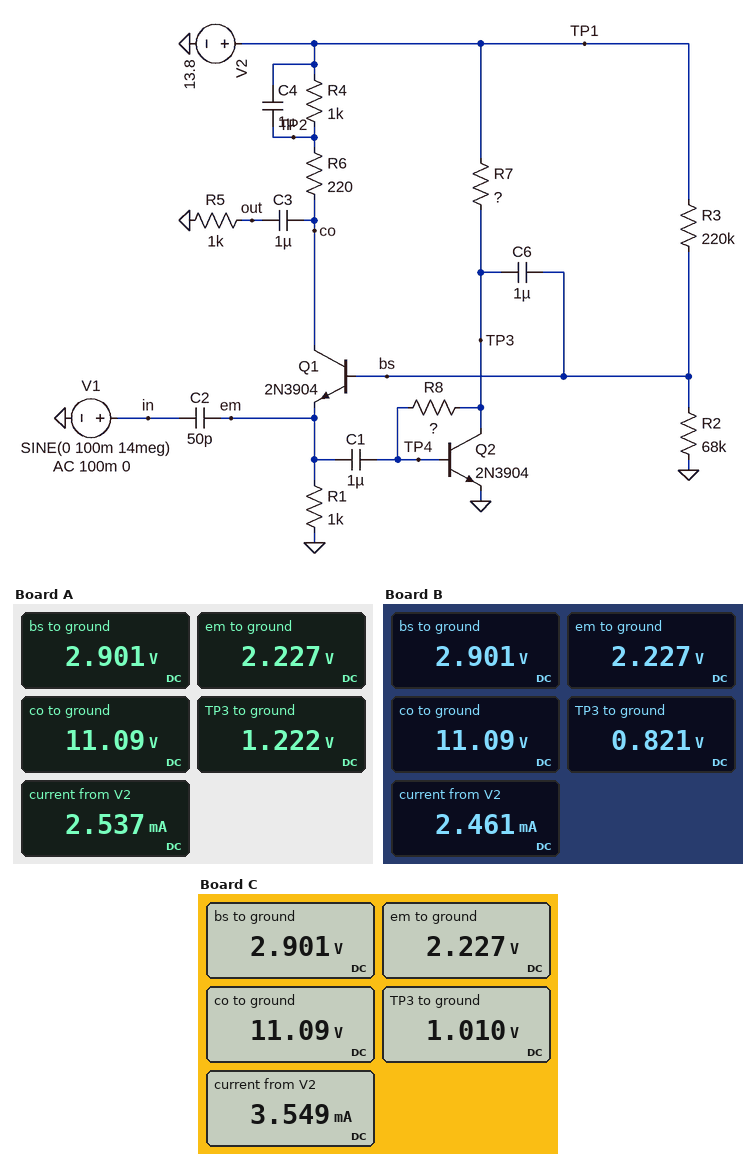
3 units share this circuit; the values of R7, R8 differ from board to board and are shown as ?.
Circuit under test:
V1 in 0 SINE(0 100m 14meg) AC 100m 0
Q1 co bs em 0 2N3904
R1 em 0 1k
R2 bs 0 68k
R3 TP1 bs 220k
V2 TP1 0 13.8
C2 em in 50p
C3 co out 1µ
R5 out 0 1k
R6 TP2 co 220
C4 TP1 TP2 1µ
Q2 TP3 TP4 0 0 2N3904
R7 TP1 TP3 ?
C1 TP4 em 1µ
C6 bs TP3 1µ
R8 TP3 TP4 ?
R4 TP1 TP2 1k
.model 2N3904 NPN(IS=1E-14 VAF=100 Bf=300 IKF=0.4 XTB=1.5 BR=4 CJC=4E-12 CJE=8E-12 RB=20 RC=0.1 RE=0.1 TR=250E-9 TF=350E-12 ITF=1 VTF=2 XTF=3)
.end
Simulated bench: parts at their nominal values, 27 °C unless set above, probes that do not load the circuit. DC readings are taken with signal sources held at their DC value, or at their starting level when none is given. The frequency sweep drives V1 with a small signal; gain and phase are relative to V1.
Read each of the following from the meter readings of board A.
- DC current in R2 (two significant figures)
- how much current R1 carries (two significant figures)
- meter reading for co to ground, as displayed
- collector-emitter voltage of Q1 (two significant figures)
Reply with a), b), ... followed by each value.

a) 43 µA
b) 2.2 mA
c) 11.09 V
d) 8.9 V
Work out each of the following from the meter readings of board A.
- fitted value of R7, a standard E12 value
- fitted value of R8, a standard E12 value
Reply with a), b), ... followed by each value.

a) 47 kΩ
b) 680 kΩ
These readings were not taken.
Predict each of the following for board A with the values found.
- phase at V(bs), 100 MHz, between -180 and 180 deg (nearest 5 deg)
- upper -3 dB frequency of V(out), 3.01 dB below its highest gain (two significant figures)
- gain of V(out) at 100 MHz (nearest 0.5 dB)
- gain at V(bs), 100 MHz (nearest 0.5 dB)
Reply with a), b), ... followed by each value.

a) 35 deg
b) 75 MHz
c) 11.5 dB
d) 1.0 dB
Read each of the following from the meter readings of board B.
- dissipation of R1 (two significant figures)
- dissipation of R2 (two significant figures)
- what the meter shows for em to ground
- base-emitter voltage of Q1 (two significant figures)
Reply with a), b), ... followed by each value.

a) 5.0 mW
b) 120 µW
c) 2.227 V
d) 670 mV
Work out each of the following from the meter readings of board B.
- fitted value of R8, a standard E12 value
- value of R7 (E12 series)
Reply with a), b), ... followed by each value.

a) 330 kΩ
b) 68 kΩ
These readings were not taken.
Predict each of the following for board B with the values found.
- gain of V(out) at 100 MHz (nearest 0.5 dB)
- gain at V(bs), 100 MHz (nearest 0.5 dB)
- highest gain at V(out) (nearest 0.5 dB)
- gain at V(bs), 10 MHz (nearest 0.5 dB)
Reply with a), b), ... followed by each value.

a) 6.5 dB
b) -0.5 dB
c) 21.0 dB
d) -27.5 dB
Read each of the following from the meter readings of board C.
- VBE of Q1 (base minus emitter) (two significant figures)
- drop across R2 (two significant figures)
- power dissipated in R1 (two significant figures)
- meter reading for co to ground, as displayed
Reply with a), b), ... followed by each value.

a) 670 mV
b) 2.9 V
c) 5.0 mW
d) 11.09 V
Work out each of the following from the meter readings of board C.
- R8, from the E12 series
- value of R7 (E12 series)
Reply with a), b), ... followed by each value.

a) 82 kΩ
b) 10 kΩ
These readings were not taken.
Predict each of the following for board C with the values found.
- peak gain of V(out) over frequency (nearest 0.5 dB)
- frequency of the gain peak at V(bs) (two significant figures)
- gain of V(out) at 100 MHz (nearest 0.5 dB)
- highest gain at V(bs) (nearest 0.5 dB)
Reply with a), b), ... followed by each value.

a) 28.5 dB
b) 130 MHz
c) 21.5 dB
d) 10.0 dB
